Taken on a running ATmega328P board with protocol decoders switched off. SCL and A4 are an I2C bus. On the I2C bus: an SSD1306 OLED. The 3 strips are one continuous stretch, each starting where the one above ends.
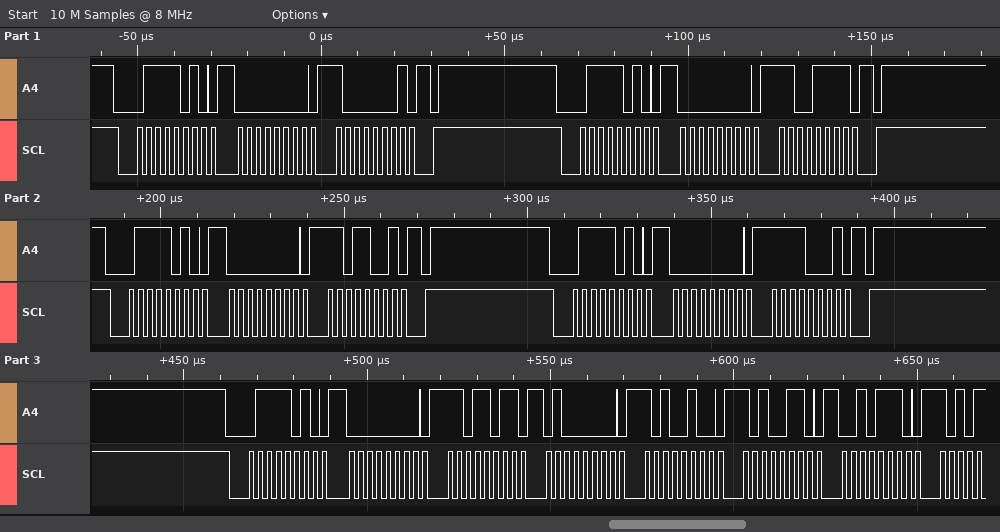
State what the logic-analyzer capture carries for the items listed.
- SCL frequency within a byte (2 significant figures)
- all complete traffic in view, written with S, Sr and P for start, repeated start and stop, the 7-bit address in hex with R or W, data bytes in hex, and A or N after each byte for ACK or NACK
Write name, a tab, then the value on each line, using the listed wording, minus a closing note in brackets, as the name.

SCL frequency within a byte	400 kHz
all complete traffic in view, written with S, Sr and P for start, repeated start and stop, the 7-bit address in hex with R or W, data bytes in hex, and A or N after each byte for ACK or NACK	S 3DW A 00 A 81 A P S 3DW A 00 A CF A P S 3DW A 00 A D9 A P S 3DW A 00 A F1 A P S 3DW A 00 A DB A 40 A A4 A A6 A 2E A
